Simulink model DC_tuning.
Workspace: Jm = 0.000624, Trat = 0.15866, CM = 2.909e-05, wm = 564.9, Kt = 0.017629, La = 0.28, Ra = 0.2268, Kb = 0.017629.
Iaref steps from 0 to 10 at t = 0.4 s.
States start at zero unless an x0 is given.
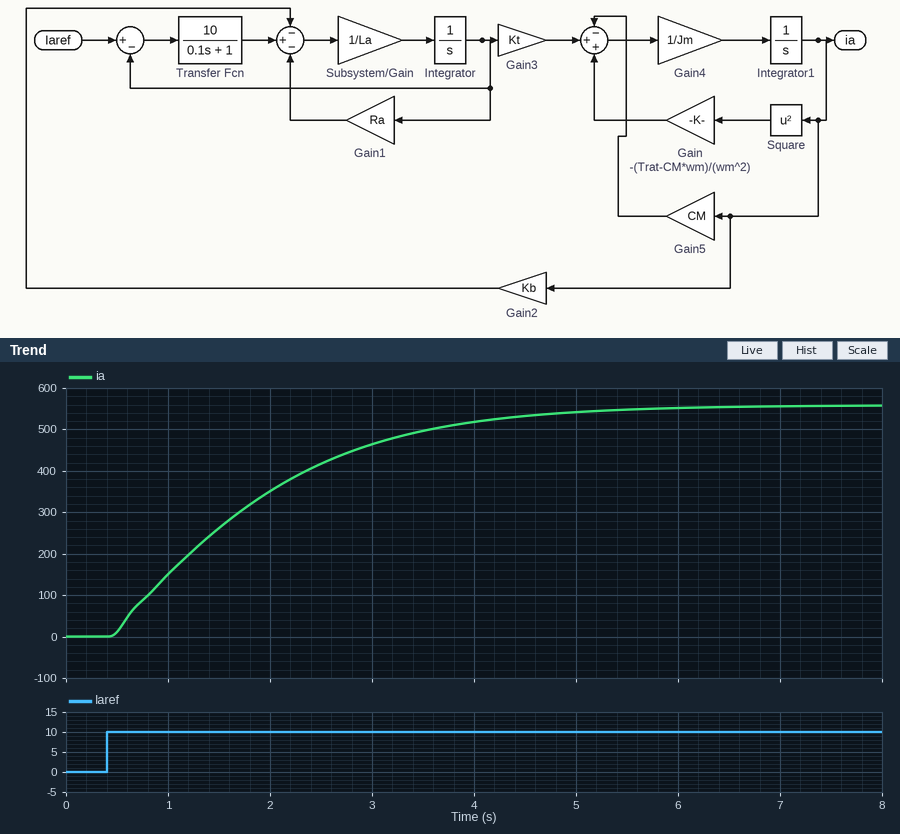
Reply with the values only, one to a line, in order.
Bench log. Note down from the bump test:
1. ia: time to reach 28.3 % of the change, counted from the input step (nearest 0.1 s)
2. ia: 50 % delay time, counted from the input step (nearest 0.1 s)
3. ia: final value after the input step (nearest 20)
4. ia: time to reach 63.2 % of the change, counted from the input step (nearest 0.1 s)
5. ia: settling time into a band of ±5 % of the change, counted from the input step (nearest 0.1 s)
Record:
0.6 s
1.2 s
560
1.6 s
4.0 s
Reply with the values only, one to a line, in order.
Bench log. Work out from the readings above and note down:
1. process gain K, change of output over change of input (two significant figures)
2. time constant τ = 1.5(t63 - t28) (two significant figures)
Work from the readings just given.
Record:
56
1.5 s
